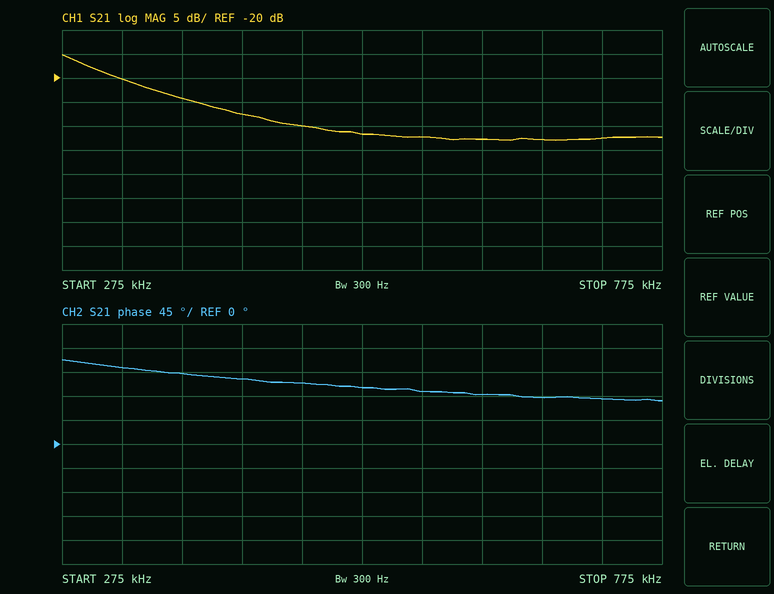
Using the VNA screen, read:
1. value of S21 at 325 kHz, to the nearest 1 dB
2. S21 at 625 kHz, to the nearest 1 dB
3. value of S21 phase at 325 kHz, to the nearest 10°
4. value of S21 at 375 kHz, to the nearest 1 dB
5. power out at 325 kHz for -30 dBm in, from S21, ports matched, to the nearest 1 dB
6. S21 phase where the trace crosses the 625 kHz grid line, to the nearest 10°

-20 dB
-33 dB
140°
-24 dB
-50 dBm
90°
